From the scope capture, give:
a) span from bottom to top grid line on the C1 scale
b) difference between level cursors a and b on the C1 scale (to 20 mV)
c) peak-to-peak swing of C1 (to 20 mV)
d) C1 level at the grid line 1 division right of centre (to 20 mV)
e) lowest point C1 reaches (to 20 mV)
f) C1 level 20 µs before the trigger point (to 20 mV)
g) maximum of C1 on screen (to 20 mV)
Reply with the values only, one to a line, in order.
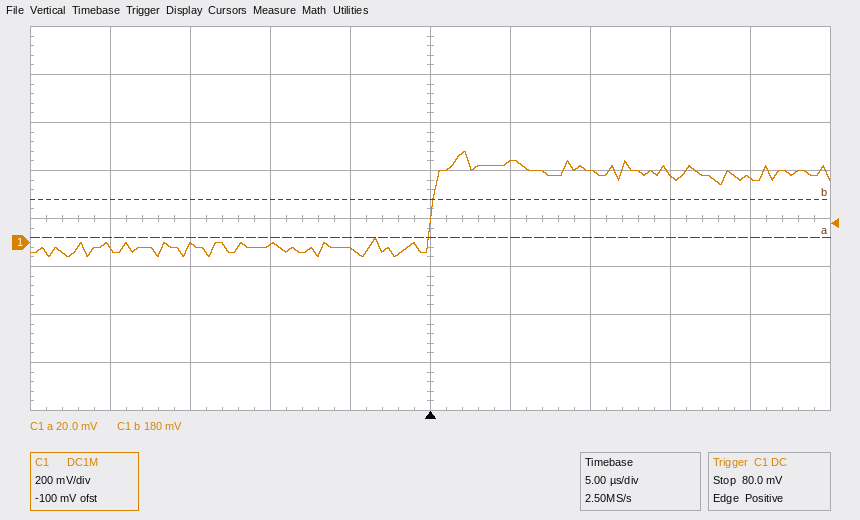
1.6 V
160 mV
440 mV
340 mV
-60 mV
-20 mV
380 mV
